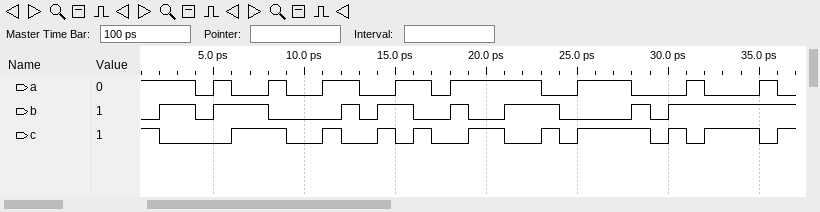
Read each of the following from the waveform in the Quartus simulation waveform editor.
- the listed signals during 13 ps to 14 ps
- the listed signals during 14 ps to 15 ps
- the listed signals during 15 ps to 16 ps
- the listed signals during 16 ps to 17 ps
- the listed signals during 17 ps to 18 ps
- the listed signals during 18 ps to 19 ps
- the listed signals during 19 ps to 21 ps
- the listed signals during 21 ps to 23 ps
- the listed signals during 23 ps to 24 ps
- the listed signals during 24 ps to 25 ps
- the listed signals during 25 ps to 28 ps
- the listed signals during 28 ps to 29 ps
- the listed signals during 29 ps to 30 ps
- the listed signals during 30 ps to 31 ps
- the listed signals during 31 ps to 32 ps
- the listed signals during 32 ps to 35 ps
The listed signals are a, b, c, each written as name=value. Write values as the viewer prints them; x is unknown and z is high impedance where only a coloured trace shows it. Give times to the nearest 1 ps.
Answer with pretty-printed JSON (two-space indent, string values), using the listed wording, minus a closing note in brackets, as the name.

{
  "the listed signals during 13 ps to 14 ps": "a=0, b=0, c=0",
  "the listed signals during 14 ps to 15 ps": "a=0, b=1, c=1",
  "the listed signals during 15 ps to 16 ps": "a=1, b=1, c=0",
  "the listed signals during 16 ps to 17 ps": "a=1, b=0, c=1",
  "the listed signals during 17 ps to 18 ps": "a=0, b=0, c=0",
  "the listed signals during 18 ps to 19 ps": "a=1, b=1, c=0",
  "the listed signals during 19 ps to 21 ps": "a=1, b=0, c=1",
  "the listed signals during 21 ps to 23 ps": "a=1, b=1, c=0",
  "the listed signals during 23 ps to 24 ps": "a=0, b=1, c=1",
  "the listed signals during 24 ps to 25 ps": "a=0, b=0, c=0",
  "the listed signals during 25 ps to 28 ps": "a=1, b=0, c=1",
  "the listed signals during 28 ps to 29 ps": "a=0, b=1, c=1",
  "the listed signals during 29 ps to 30 ps": "a=0, b=0, c=0",
  "the listed signals during 30 ps to 31 ps": "a=0, b=1, c=1",
  "the listed signals during 31 ps to 32 ps": "a=1, b=1, c=0",
  "the listed signals during 32 ps to 35 ps": "a=0, b=1, c=1"
}
